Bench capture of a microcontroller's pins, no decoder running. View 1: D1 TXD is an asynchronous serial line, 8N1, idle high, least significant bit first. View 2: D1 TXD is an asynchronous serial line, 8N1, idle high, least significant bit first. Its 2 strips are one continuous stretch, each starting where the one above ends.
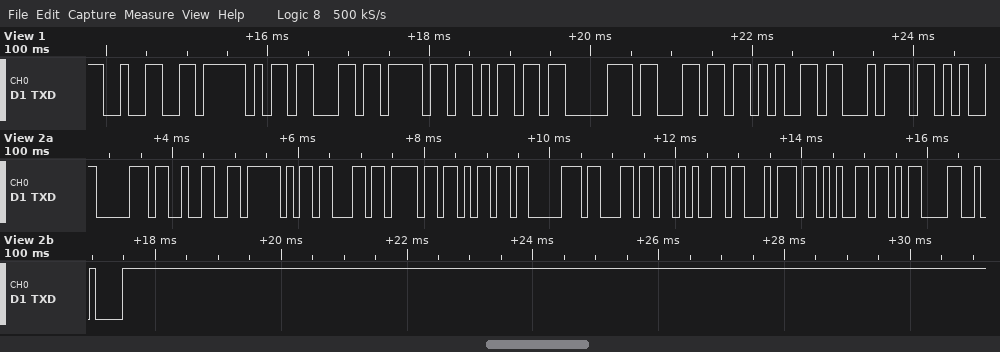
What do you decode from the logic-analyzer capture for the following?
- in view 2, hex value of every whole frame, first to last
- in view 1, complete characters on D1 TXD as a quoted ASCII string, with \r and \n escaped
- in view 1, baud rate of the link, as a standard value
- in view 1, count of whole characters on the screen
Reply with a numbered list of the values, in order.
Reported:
1. 70 32 5F 63 6F 6D 70 6C 65 74 65 0D 0A
2. "2_complet"
3. 9600 baud
4. 9
